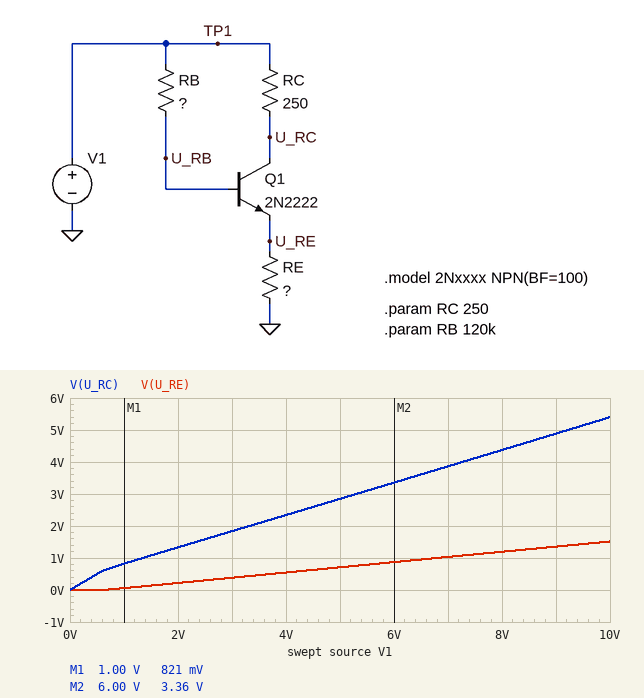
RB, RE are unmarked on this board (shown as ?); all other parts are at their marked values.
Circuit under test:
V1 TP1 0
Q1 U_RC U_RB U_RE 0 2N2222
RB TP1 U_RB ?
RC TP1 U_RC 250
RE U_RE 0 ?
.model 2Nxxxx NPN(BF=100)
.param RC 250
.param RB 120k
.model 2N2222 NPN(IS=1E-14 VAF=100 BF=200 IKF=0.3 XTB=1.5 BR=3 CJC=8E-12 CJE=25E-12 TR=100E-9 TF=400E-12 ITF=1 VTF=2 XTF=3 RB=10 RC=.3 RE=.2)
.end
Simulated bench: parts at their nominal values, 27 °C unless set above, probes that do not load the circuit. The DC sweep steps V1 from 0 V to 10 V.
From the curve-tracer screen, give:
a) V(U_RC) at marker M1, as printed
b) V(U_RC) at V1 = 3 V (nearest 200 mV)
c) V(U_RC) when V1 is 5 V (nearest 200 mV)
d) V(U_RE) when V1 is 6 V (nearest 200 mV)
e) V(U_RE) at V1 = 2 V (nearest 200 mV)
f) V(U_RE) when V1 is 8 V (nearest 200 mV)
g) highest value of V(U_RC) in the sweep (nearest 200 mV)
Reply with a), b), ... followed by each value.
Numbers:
a) 821 mV
b) 1.8 V
c) 2.8 V
d) 800 mV
e) 200 mV
f) 1.2 V
g) 5.4 V
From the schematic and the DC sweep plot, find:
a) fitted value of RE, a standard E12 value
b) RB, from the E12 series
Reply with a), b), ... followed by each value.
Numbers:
a) 82 Ω
b) 82 kΩ
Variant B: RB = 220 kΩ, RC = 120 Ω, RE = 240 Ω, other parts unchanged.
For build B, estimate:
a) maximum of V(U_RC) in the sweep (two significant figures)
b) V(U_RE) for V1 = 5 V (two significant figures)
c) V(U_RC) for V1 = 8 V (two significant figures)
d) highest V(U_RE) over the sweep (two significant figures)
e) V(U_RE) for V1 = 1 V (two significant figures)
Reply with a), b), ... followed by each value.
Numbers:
a) 9.1 V
b) 790 mV
c) 7.3 V
d) 1.7 V
e) 68 mV
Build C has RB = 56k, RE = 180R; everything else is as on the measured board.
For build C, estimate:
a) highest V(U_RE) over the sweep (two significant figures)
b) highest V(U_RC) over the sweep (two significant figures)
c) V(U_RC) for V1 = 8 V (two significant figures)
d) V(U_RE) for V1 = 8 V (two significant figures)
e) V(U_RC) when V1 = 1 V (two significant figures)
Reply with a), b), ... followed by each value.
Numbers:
a) 3.5 V
b) 5.1 V
c) 4.2 V
d) 2.8 V
e) 810 mV
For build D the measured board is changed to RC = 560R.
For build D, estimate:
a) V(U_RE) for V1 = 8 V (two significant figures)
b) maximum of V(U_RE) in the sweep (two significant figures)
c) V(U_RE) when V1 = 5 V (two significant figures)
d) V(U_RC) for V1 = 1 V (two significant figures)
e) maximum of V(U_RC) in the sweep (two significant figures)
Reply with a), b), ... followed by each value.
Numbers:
a) 1.0 V
b) 1.3 V
c) 620 mV
d) 600 mV
e) 1.4 V
